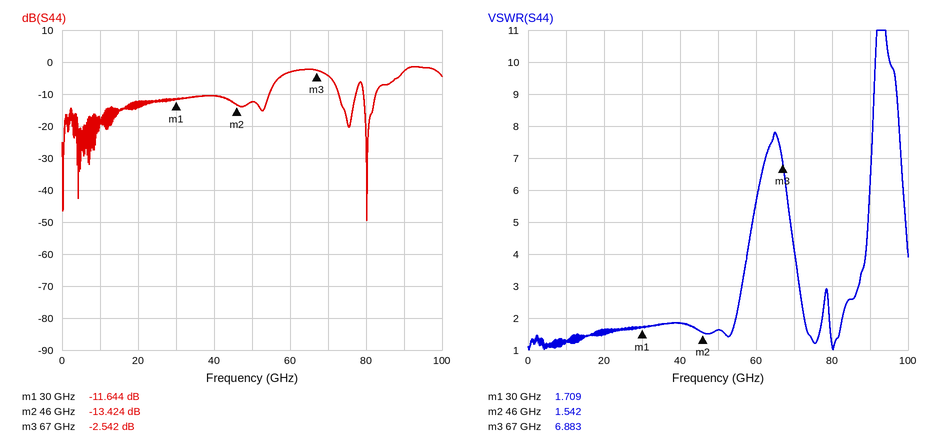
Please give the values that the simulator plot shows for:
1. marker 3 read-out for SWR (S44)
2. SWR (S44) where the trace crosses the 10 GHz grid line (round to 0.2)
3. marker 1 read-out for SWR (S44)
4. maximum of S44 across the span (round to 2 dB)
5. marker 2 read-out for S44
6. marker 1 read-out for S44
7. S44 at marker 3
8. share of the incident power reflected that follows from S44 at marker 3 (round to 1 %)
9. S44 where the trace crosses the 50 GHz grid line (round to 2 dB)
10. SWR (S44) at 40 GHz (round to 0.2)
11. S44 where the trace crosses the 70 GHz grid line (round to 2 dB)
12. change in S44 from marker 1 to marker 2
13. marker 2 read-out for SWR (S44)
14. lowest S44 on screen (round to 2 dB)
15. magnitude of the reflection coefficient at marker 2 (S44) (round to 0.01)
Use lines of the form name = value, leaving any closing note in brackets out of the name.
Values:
marker 3 read-out for SWR = 6.883
SWR (S44) where the trace crosses the 10 GHz grid line = 1.2
marker 1 read-out for SWR = 1.709
maximum of S44 across the span = -2 dB
marker 2 read-out for S44 = -13.424 dB
marker 1 read-out for S44 = -11.644 dB
S44 at marker 3 = -2.542 dB
share of the incident power reflected that follows from S44 at marker 3 = 56 %
S44 where the trace crosses the 50 GHz grid line = -12 dB
SWR (S44) at 40 GHz = 1.8
S44 where the trace crosses the 70 GHz grid line = -4 dB
change in S44 from marker 1 to marker 2 = -1.780 dB
marker 2 read-out for SWR = 1.542
lowest S44 on screen = -50 dB
magnitude of the reflection coefficient at marker 2 (S44) = 0.21
